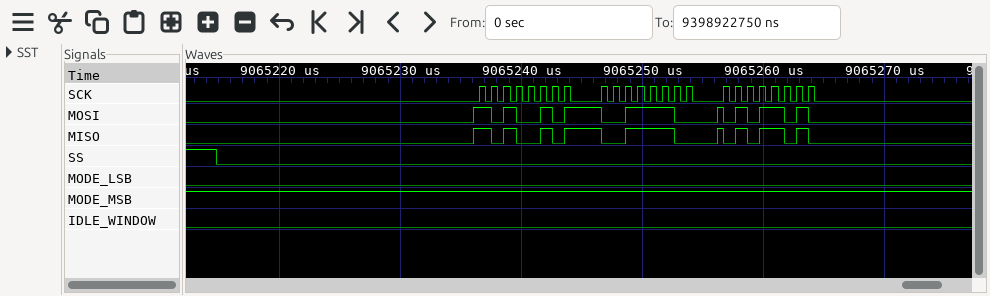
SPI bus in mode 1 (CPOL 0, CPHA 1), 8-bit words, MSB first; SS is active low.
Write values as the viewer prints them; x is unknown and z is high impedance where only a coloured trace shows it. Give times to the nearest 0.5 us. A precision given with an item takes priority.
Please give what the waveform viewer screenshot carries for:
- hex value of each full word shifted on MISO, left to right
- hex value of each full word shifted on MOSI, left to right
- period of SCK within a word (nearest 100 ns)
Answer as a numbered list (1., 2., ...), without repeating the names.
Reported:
1. A5, 3C, 5A
2. A5, 3C, 5A
3. 1000 ns
